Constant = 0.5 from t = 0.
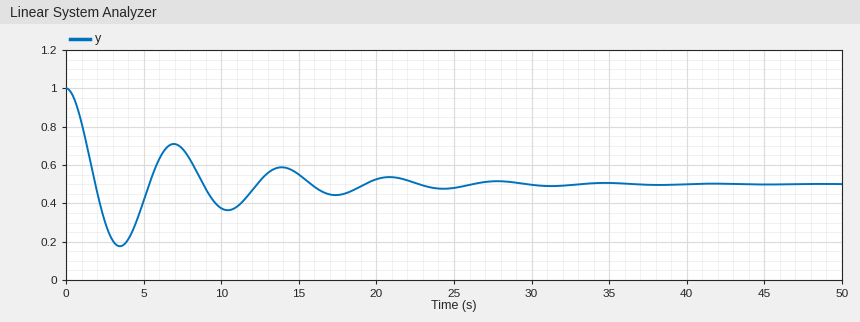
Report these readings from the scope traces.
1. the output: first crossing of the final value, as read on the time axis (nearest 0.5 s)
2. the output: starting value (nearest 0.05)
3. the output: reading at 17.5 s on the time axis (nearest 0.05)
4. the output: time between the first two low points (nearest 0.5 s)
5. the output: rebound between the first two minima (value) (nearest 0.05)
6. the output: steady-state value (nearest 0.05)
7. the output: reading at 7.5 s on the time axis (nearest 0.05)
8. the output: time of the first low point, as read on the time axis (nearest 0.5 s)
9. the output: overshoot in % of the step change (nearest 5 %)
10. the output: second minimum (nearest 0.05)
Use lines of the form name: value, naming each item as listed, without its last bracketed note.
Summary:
the output: first crossing of the final value, as read on the time axis: 2.0 s
the output: starting value: 1.00
the output: reading at 17.5 s on the time axis: 0.45
the output: time between the first two low points: 7.0 s
the output: rebound between the first two minima (value): 0.70
the output: steady-state value: 0.50
the output: reading at 7.5 s on the time axis: 0.70
the output: time of the first low point, as read on the time axis: 3.5 s
the output: overshoot in % of the step change: 65 %
the output: second minimum: 0.35
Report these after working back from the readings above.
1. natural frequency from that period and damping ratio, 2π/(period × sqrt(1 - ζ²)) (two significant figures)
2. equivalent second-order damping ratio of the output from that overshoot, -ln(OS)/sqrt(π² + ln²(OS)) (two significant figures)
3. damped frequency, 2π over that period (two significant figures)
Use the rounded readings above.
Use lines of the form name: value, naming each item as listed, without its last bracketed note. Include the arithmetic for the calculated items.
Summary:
natural frequency from that period and damping ratio, 2π/(period × sqrt(1 - ζ²)): 2π / (7 × sqrt(1 - 0.14²)) = 0.91 rad/s
equivalent second-order damping ratio of the output from that overshoot, -ln(OS)/sqrt(π² + ln²(OS)): ln(0.65) = -0.431; 0.431 / sqrt(9.870 + 0.186) = 0.14
damped frequency, 2π over that period: 2π / 7 = 0.90 rad/s
